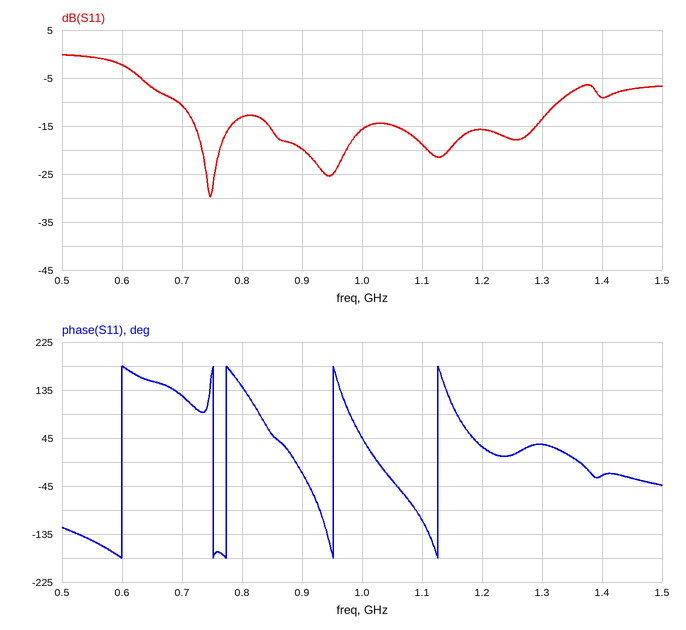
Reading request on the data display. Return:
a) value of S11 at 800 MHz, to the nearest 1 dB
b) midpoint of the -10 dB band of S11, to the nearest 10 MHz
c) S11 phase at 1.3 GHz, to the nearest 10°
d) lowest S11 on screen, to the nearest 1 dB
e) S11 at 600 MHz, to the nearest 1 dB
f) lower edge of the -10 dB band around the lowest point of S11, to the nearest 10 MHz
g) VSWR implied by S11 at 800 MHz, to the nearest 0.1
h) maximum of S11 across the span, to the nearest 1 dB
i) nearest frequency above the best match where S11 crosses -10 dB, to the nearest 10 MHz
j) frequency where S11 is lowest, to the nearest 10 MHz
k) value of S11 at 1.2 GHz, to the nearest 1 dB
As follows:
-13 dB
1.01 GHz
30°
-30 dB
-2 dB
690 MHz
1.6
0 dB
1.33 GHz
750 MHz
-16 dB
